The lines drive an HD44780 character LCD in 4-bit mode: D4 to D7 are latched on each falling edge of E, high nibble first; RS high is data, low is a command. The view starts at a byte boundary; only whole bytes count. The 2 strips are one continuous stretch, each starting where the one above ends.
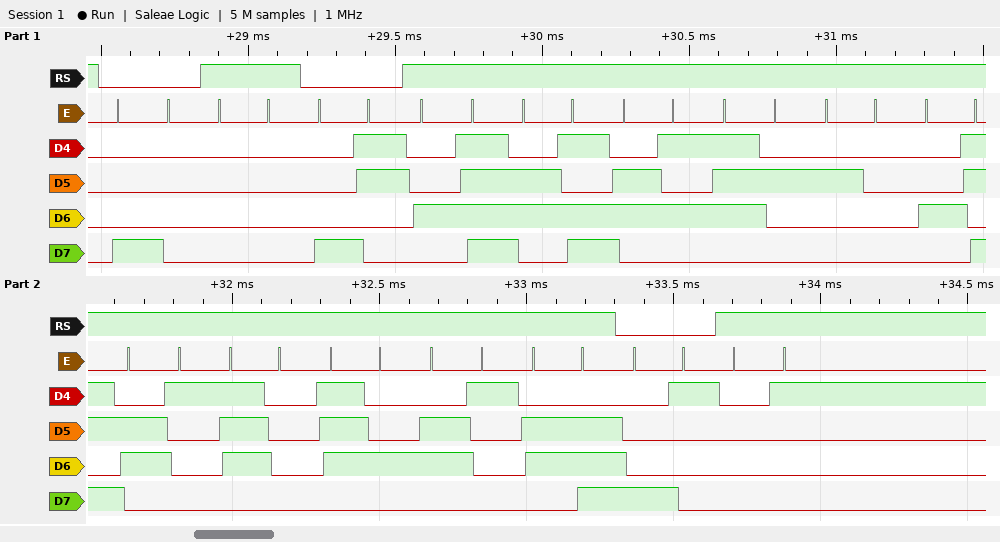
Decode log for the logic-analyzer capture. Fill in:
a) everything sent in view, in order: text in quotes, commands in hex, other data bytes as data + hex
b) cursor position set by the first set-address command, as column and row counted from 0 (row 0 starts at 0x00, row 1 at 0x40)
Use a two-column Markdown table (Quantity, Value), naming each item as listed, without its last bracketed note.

| Quantity | Value |
|---|---|
| everything sent in view, in order: text in quotes, commands in hex, other data bytes as data + hex | 0x80 data 00 0x83 "Omer Kaptan" 0x81 data 01 |
| cursor position set by the first set-address command, as column and row counted from 0 | column 0, row 0 |
